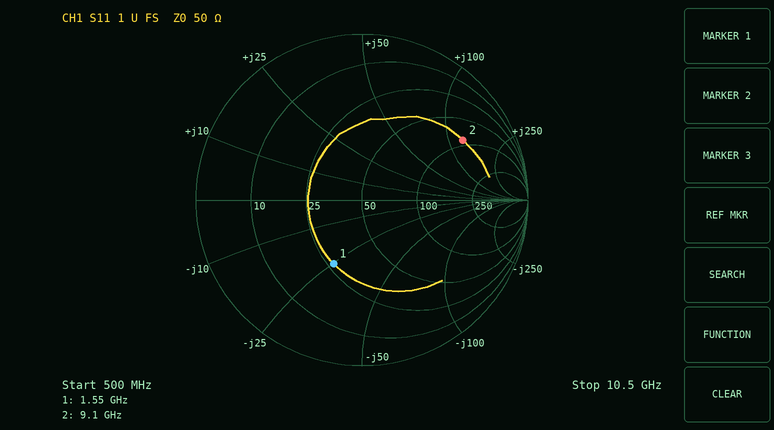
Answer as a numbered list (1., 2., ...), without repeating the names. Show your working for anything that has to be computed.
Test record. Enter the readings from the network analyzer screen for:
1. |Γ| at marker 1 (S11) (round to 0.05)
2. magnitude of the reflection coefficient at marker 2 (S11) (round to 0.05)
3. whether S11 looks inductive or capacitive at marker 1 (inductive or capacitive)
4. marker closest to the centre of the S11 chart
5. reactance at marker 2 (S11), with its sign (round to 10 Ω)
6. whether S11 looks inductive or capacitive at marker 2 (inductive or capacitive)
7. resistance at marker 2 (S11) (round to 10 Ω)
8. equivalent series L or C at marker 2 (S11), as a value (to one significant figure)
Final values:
1. 0.40
2. 0.70
3. capacitive
4. marker 1
5. +130 Ω
6. inductive
7. 90 Ω
8. L = 130 Ω/(2π × 9.1 GHz) ≈ 2 nH
